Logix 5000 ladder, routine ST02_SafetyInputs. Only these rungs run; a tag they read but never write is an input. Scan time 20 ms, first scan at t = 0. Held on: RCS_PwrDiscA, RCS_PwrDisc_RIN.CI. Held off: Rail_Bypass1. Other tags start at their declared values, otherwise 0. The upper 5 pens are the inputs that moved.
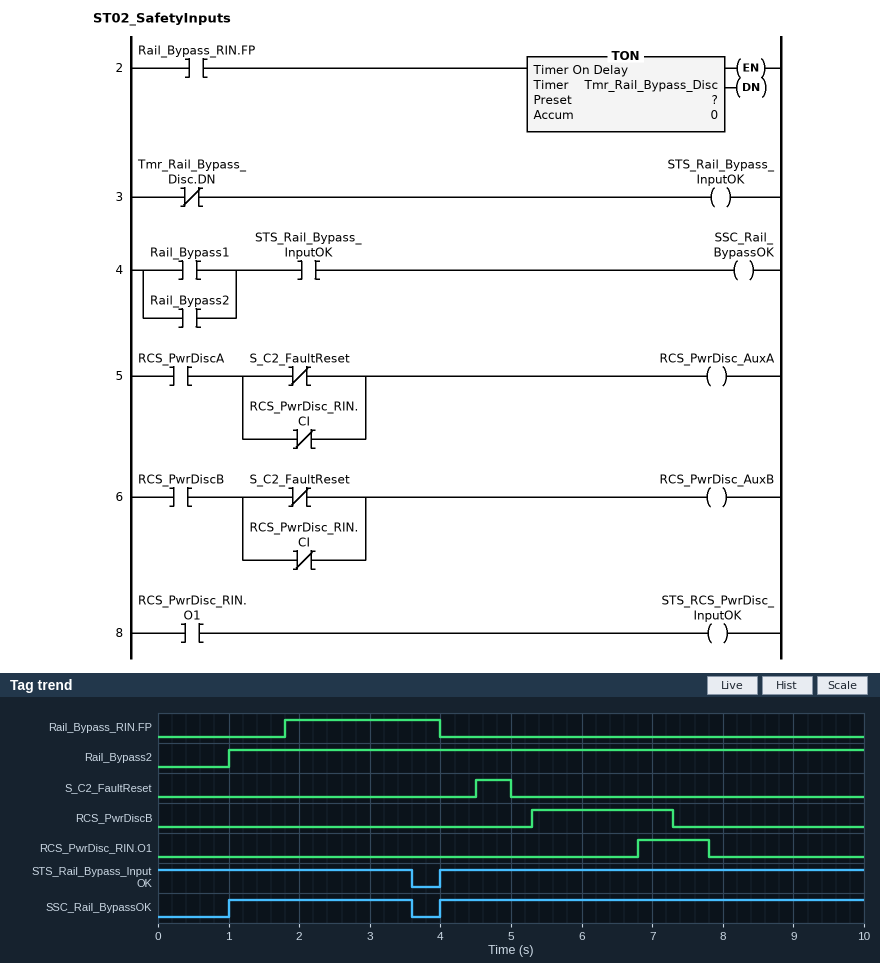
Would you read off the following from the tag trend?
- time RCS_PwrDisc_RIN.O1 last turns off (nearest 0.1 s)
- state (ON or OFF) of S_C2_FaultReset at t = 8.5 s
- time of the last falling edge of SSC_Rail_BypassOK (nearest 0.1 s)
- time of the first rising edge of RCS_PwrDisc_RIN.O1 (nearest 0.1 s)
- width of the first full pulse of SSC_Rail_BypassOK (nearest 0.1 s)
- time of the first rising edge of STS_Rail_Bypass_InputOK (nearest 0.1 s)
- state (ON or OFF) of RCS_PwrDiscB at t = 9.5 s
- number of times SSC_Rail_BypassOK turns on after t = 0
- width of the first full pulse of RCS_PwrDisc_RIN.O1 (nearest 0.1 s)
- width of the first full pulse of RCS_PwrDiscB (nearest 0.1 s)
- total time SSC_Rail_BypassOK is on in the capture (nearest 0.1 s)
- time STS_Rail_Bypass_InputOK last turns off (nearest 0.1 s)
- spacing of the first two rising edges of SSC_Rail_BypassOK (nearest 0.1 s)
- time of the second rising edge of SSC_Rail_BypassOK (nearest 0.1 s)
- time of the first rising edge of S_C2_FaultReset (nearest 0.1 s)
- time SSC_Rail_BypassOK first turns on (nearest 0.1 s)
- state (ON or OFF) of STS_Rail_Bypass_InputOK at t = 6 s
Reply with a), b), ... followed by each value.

a) 7.8 s
b) OFF
c) 3.6 s
d) 6.8 s
e) 2.6 s
f) 4.0 s
g) OFF
h) 2
i) 1.0 s
j) 2.0 s
k) 8.6 s
l) 3.6 s
m) 3.0 s
n) 4.0 s
o) 4.5 s
p) 1.0 s
q) ON
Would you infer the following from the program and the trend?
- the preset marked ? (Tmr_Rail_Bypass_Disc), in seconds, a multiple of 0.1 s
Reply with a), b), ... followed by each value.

a) 1.8 s
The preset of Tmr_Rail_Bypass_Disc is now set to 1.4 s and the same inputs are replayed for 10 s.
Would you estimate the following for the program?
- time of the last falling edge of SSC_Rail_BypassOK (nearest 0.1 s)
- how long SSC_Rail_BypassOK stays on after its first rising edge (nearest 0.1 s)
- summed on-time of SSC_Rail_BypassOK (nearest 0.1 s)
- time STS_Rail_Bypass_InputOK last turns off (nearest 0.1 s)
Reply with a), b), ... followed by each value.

a) 3.2 s
b) 2.2 s
c) 8.2 s
d) 3.2 s
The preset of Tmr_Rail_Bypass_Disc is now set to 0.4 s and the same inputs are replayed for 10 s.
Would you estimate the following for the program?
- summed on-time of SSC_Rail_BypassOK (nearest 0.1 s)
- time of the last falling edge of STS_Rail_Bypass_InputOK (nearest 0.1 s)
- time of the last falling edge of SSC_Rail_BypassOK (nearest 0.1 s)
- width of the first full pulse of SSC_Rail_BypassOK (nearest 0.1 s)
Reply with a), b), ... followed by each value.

a) 7.2 s
b) 2.2 s
c) 2.2 s
d) 1.2 s
